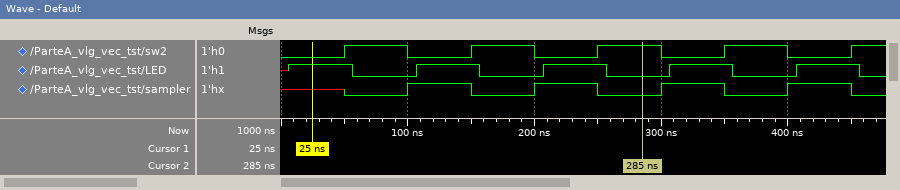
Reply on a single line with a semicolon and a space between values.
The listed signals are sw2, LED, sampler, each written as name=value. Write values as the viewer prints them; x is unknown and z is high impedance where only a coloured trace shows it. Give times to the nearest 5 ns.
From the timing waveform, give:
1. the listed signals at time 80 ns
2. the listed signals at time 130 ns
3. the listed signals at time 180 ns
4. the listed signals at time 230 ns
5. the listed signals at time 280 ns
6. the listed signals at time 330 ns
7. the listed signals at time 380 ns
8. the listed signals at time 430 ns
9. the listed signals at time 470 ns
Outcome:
sw2=1, LED=0, sampler=0; sw2=0, LED=1, sampler=1; sw2=1, LED=0, sampler=0; sw2=0, LED=1, sampler=1; sw2=1, LED=0, sampler=0; sw2=0, LED=1, sampler=1; sw2=1, LED=0, sampler=0; sw2=0, LED=1, sampler=1; sw2=1, LED=0, sampler=0
